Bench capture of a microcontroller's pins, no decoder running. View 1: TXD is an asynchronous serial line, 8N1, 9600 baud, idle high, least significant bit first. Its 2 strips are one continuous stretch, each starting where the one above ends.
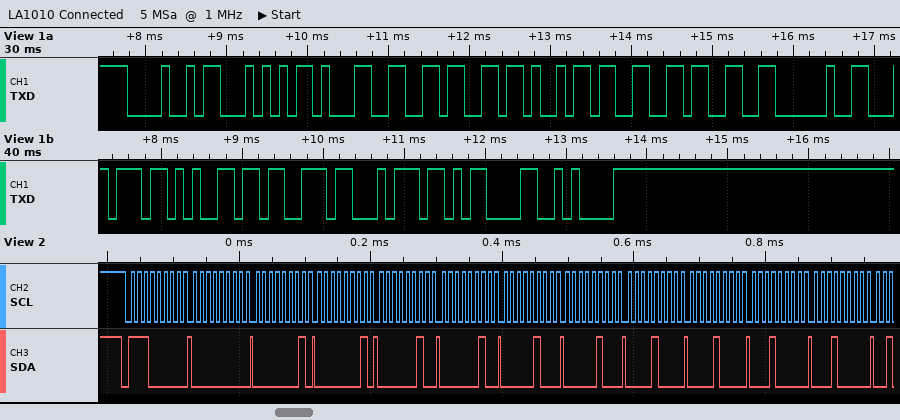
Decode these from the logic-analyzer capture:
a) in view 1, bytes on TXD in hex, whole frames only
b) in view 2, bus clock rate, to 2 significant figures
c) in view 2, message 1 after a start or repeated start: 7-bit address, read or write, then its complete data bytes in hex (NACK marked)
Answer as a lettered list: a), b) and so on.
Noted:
a) 48 54 31 36 4B 33 33 20 74 65 73 74 0D 0A
b) 100 kHz
c) 0x70 write: 00 01 01 02 02 04 04 08 08 10 10
